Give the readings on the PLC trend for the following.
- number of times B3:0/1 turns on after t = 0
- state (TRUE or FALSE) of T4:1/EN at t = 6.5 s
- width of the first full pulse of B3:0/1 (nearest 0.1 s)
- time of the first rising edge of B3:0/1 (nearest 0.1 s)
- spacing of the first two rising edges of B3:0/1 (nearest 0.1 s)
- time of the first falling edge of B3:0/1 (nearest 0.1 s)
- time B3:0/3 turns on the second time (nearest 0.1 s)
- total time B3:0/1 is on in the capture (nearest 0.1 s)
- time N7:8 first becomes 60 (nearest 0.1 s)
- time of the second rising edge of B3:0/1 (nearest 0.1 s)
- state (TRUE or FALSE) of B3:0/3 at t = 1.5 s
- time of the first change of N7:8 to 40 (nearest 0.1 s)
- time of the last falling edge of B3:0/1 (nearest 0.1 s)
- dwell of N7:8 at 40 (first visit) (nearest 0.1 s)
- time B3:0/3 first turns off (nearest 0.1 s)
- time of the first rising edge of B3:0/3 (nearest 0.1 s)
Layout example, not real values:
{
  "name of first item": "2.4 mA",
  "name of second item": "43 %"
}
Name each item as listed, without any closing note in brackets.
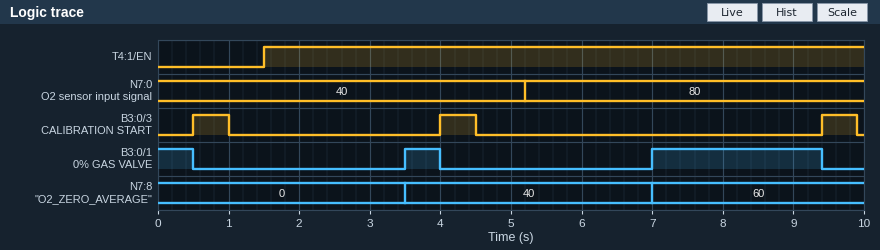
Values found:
{
  "number of times B3:0/1 turns on after t = 0": "2",
  "state (TRUE or FALSE) of T4:1/EN at t = 6.5 s": "TRUE",
  "width of the first full pulse of B3:0/1": "0.5 s",
  "time of the first rising edge of B3:0/1": "3.5 s",
  "spacing of the first two rising edges of B3:0/1": "3.5 s",
  "time of the first falling edge of B3:0/1": "0.5 s",
  "time B3:0/3 turns on the second time": "4.0 s",
  "total time B3:0/1 is on in the capture": "3.4 s",
  "time N7:8 first becomes 60": "7.0 s",
  "time of the second rising edge of B3:0/1": "7.0 s",
  "state (TRUE or FALSE) of B3:0/3 at t = 1.5 s": "FALSE",
  "time of the first change of N7:8 to 40": "3.5 s",
  "time of the last falling edge of B3:0/1": "9.4 s",
  "dwell of N7:8 at 40 (first visit)": "3.5 s",
  "time B3:0/3 first turns off": "1.0 s",
  "time of the first rising edge of B3:0/3": "0.5 s"
}
